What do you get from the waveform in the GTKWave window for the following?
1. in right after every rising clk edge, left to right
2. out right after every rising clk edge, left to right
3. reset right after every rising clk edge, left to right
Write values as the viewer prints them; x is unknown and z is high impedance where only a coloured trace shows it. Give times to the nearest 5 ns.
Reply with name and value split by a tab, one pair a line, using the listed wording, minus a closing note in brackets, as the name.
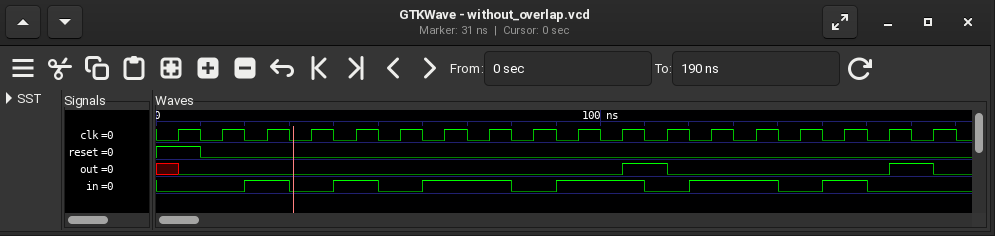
in right after every rising clk edge, left to right	0 0 1 0 1 0 1 1 0 1 1 0 1 1 0 1 0 0
out right after every rising clk edge, left to right	0 0 0 0 0 0 0 0 0 0 1 0 0 0 0 0 1 0
reset right after every rising clk edge, left to right	1 0 0 0 0 0 0 0 0 0 0 0 0 0 0 0 0 0
